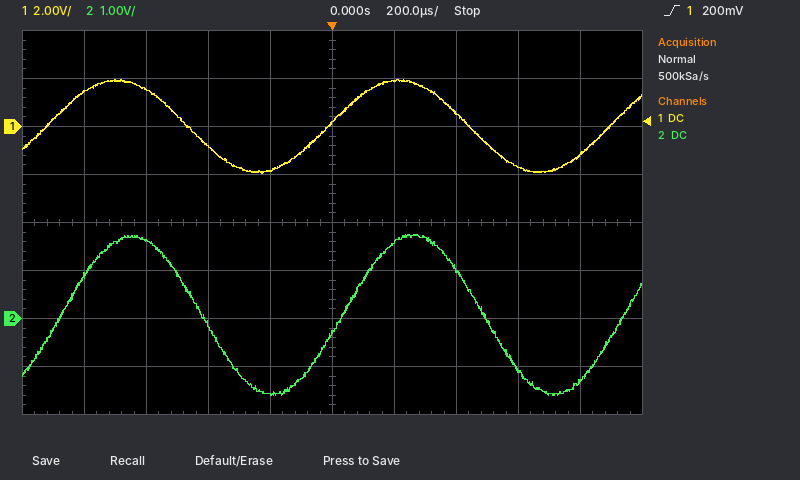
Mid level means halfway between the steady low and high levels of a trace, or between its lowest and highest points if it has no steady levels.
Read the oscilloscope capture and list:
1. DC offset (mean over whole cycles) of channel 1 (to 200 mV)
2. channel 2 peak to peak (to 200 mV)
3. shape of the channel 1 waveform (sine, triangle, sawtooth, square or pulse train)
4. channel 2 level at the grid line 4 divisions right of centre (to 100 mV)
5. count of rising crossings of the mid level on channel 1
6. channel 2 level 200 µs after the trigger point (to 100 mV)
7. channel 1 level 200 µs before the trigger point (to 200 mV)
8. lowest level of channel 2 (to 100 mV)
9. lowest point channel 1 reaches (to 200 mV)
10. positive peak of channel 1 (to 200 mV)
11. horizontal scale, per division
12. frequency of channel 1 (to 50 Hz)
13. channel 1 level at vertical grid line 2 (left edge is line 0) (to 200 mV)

0.0 V
3.4 V
sine
-1.3 V
3
1.6 V
-1.8 V
-1.6 V
-2.0 V
2.0 V
200 µs
1.10 kHz
1.6 V
